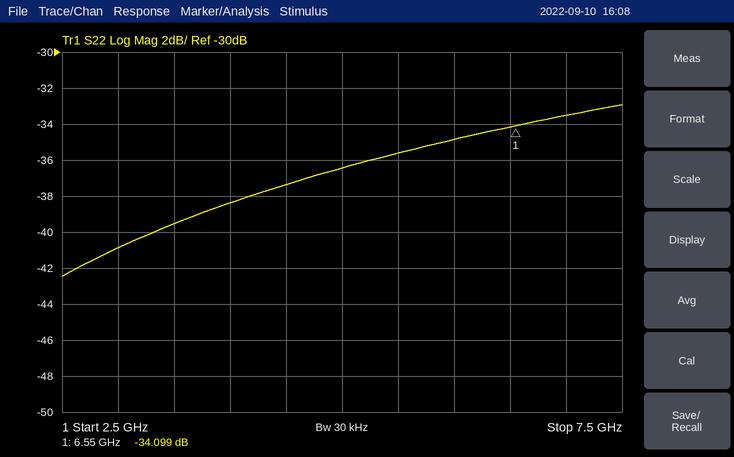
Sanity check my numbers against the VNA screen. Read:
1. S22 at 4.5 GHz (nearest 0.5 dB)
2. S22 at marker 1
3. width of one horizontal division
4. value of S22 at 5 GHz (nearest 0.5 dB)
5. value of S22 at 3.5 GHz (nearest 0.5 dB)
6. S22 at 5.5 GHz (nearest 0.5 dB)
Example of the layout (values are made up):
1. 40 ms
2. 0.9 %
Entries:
1. -37.5 dB
2. -34.099 dB
3. 500 MHz
4. -36.5 dB
5. -39.5 dB
6. -35.5 dB
